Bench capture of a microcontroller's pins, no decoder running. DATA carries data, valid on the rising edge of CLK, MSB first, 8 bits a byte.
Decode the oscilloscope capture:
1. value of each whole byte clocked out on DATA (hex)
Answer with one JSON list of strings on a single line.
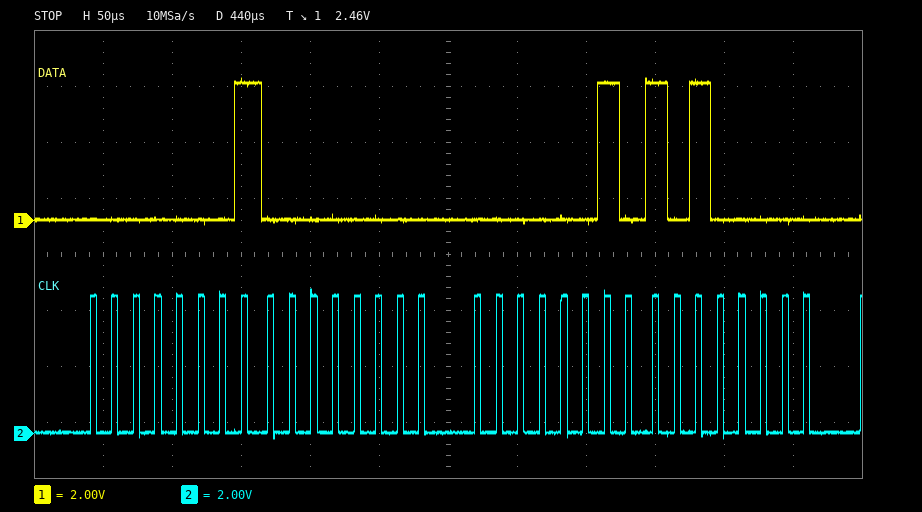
["01 00 02 A0"]
